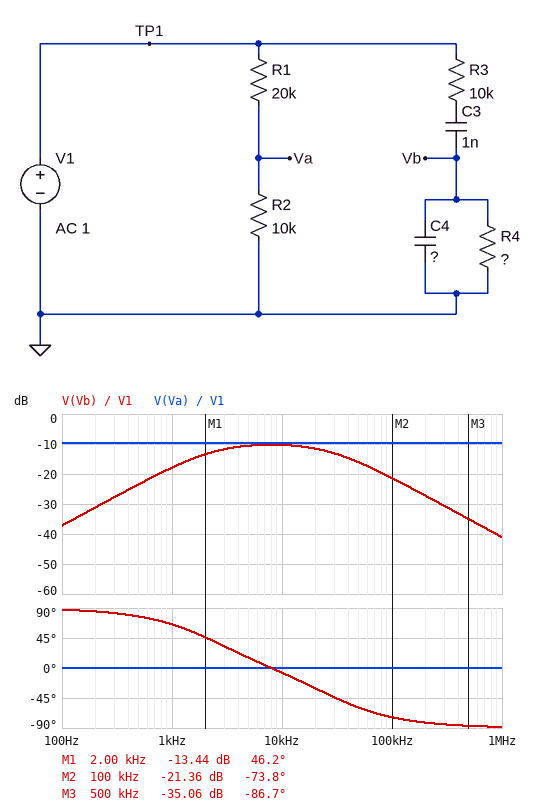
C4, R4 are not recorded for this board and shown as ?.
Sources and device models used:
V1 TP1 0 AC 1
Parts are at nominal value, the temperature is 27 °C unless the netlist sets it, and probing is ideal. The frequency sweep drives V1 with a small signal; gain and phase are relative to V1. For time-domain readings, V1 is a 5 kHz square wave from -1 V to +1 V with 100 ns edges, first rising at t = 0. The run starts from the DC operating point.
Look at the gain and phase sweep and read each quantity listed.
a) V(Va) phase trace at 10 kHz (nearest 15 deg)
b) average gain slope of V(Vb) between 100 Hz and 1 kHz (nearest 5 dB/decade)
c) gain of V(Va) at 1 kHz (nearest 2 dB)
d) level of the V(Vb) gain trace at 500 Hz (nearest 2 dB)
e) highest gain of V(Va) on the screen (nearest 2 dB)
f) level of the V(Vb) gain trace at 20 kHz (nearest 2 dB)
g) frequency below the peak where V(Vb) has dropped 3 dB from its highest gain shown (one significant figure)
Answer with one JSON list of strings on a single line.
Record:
["0 deg", "20 dB/decade", "-10 dB", "-24 dB", "-10 dB", "-12 dB", "2 kHz"]
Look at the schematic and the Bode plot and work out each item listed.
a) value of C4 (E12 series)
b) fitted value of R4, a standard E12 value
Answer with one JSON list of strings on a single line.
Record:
["1.8 nF", "22 kΩ"]
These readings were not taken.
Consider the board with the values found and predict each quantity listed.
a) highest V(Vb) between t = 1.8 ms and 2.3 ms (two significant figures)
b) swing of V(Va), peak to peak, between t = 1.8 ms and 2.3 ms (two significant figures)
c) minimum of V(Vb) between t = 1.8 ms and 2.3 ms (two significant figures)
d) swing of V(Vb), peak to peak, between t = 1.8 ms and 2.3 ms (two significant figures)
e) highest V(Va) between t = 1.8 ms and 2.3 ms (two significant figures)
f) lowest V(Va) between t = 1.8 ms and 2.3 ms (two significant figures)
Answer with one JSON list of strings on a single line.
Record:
["420 mV", "670 mV", "-420 mV", "850 mV", "330 mV", "-330 mV"]
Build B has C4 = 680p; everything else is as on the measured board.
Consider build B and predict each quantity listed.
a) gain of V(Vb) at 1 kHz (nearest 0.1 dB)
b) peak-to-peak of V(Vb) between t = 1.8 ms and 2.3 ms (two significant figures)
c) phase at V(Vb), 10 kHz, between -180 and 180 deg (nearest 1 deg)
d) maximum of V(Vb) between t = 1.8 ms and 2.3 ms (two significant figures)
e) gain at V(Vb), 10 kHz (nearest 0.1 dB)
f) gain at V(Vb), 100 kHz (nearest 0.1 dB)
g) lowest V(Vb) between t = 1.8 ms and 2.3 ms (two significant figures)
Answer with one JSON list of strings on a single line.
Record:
["-17.5 dB", "1.5 V", "8 deg", "730 mV", "-6.7 dB", "-13.5 dB", "-730 mV"]
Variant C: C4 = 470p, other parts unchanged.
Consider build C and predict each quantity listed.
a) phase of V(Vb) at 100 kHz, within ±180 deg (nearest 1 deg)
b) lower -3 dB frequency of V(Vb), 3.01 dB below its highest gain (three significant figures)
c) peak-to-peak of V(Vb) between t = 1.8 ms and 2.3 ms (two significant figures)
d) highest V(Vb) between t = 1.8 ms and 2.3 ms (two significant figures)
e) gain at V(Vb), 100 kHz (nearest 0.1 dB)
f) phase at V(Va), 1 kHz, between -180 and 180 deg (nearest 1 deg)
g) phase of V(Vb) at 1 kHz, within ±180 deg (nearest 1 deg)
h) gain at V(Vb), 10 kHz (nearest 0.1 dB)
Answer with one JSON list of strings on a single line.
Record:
["-56 deg", "3.56 kHz", "1.7 V", "840 mV", "-10.8 dB", "0 deg", "75 deg", "-5.9 dB"]
